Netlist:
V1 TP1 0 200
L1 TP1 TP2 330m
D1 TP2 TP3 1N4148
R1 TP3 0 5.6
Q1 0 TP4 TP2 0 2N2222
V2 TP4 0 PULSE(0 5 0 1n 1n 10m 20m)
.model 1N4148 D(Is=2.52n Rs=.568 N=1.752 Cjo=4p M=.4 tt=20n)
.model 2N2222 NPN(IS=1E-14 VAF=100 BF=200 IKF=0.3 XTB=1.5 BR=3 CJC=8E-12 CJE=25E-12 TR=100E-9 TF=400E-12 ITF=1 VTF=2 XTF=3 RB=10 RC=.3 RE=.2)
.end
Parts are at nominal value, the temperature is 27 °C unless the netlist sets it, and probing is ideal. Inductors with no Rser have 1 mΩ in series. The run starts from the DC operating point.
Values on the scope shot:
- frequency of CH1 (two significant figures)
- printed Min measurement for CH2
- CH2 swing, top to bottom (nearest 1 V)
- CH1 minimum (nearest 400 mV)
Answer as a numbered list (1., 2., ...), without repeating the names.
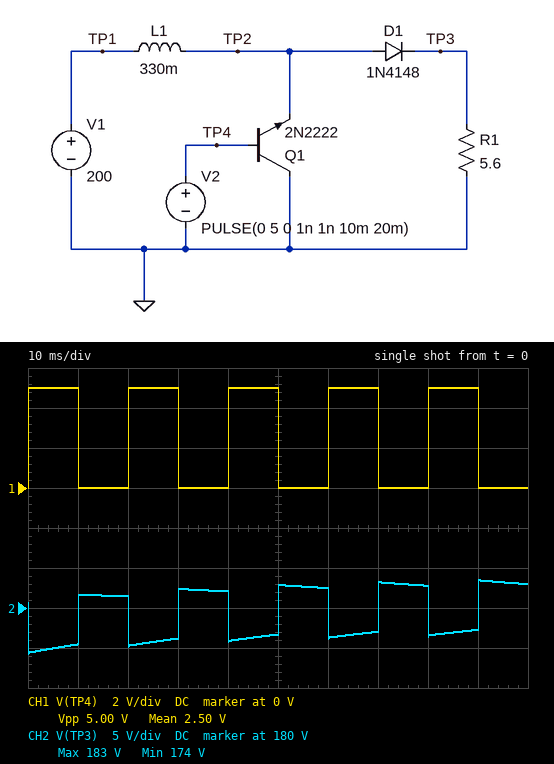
1. 50 Hz
2. 174 V
3. 9 V
4. 0 V
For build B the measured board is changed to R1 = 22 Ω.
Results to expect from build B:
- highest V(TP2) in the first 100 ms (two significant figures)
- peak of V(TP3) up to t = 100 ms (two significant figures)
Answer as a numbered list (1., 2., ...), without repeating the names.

1. 220 V
2. 210 V
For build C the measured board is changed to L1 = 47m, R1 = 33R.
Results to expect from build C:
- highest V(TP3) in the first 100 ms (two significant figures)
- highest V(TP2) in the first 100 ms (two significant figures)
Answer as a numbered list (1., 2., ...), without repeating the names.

1. 230 V
2. 240 V
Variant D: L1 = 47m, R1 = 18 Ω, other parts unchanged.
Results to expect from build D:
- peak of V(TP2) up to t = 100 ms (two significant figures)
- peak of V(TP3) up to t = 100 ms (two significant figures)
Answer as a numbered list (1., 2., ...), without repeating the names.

1. 220 V
2. 210 V
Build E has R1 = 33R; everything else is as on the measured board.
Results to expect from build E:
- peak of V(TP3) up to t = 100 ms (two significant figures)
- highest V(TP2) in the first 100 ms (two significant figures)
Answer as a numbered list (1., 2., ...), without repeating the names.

1. 220 V
2. 230 V
